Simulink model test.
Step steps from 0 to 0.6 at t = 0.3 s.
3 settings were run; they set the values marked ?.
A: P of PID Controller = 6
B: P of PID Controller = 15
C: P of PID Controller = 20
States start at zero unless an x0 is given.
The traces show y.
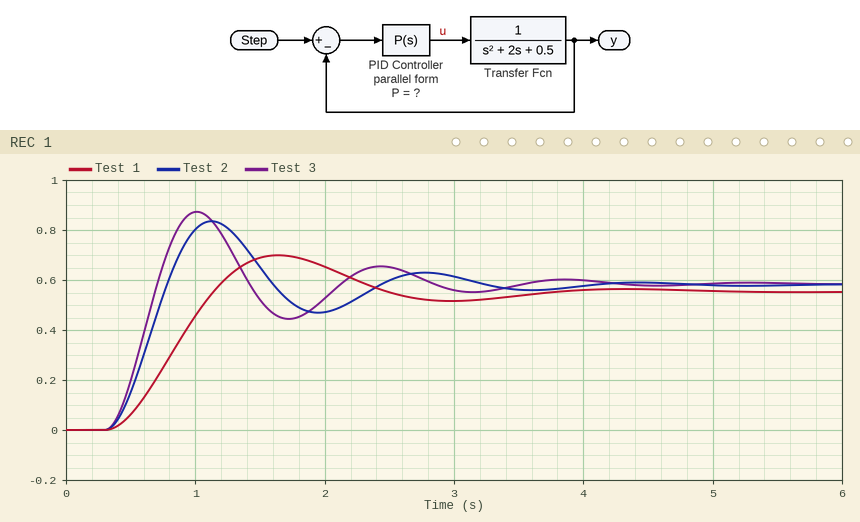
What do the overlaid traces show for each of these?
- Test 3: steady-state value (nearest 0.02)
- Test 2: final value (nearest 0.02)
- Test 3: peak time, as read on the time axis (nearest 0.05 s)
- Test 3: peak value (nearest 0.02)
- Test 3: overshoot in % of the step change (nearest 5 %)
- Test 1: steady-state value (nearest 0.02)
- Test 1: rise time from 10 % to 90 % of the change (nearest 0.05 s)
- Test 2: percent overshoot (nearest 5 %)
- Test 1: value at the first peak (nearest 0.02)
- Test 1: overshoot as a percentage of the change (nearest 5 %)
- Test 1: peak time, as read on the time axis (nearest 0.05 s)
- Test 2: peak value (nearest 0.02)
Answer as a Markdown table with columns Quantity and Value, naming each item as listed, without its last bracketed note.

| Quantity | Value |
|---|---|
| Test 3: steady-state value | 0.58 |
| Test 2: final value | 0.58 |
| Test 3: peak time, as read on the time axis | 1.00 s |
| Test 3: peak value | 0.88 |
| Test 3: overshoot in % of the step change | 50 % |
| Test 1: steady-state value | 0.56 |
| Test 1: rise time from 10 % to 90 % of the change | 0.55 s |
| Test 2: percent overshoot | 45 % |
| Test 1: value at the first peak | 0.70 |
| Test 1: overshoot as a percentage of the change | 25 % |
| Test 1: peak time, as read on the time axis | 1.65 s |
| Test 2: peak value | 0.84 |
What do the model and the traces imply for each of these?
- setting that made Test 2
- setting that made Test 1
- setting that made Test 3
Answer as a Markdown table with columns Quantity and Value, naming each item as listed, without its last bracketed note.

| Quantity | Value |
|---|---|
| setting that made Test 2 | B |
| setting that made Test 1 | A |
| setting that made Test 3 | C |
